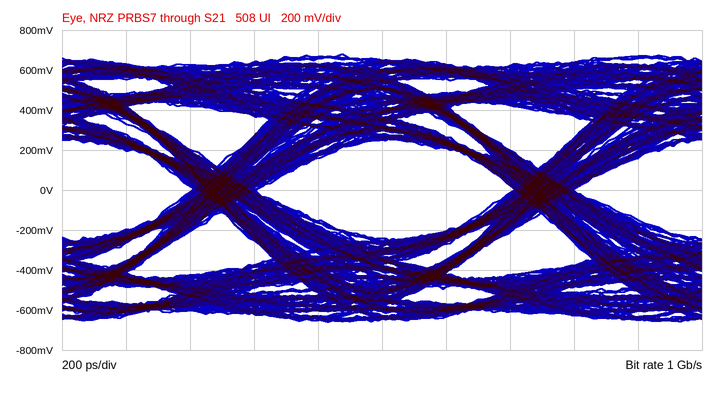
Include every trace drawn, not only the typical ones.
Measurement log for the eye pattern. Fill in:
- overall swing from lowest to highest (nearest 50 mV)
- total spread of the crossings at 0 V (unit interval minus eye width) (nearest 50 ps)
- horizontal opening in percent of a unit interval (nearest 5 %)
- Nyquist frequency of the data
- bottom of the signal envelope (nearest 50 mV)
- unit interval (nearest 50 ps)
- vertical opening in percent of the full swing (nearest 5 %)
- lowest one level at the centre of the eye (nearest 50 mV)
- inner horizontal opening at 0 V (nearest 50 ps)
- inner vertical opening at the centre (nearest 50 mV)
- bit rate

1.35 V
200 ps
80 %
500 MHz
-650 mV
1.00 ns
35 %
250 mV
800 ps
500 mV
1 Gb/s
